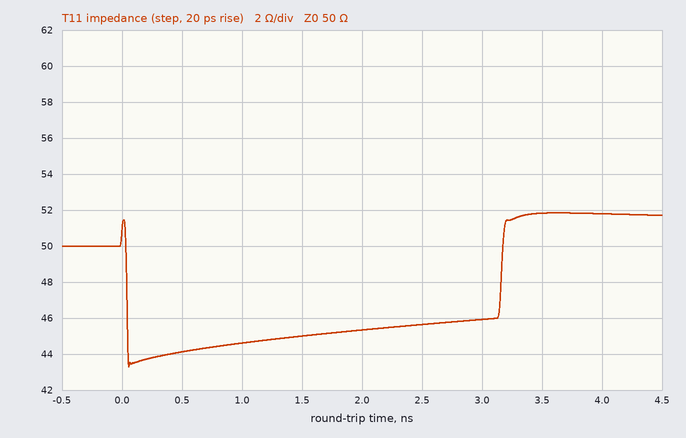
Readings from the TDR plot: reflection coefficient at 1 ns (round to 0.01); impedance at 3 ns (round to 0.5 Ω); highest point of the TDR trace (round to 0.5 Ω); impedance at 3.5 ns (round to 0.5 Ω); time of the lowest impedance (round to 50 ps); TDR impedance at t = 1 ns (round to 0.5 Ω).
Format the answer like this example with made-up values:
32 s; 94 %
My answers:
-0.06; 46.0 Ω; 52.0 Ω; 52.0 Ω; 50 ps; 44.5 Ω
